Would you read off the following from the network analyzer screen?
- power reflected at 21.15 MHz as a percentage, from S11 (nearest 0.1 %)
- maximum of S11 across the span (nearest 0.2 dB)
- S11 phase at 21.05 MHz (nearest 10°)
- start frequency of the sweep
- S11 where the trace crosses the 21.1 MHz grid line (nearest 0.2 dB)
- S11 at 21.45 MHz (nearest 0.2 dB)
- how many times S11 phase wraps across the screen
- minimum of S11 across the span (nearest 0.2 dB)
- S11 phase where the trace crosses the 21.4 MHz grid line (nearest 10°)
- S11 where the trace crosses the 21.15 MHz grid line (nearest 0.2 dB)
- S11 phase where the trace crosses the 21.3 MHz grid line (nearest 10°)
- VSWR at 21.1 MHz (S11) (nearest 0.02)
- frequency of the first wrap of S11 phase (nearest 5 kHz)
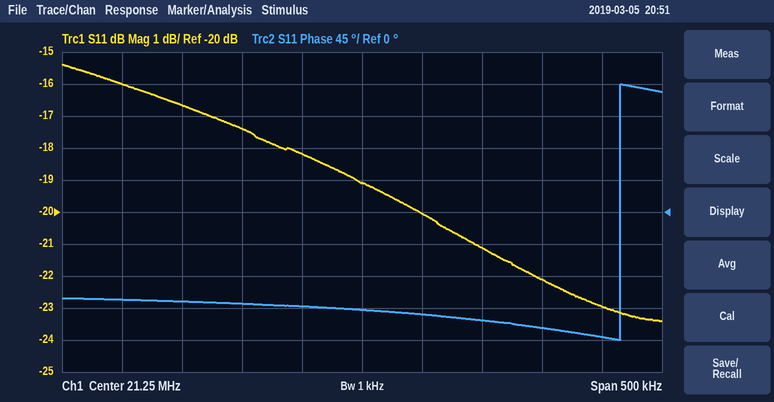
1.8 %
-15.4 dB
-120°
21 MHz
-16.6 dB
-23.0 dB
1
-23.4 dB
-160°
-17.4 dB
-140°
1.34
21.465 MHz
